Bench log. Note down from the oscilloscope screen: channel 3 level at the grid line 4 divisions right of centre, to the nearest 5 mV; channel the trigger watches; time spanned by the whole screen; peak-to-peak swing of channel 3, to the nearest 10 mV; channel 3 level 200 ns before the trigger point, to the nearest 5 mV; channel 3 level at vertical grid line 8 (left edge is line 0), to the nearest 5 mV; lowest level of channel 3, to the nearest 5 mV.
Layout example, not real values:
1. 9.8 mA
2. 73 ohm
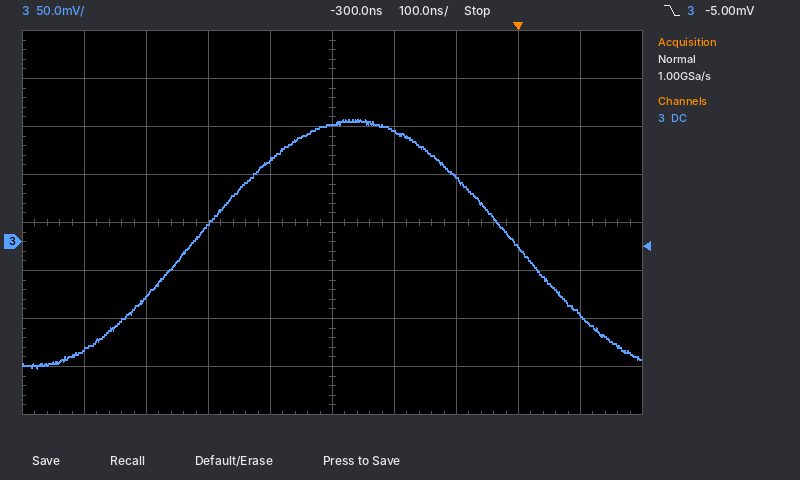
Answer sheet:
1. -75 mV
2. channel 3
3. 1 µs
4. 260 mV
5. 115 mV
6. -5 mV
7. -130 mV
